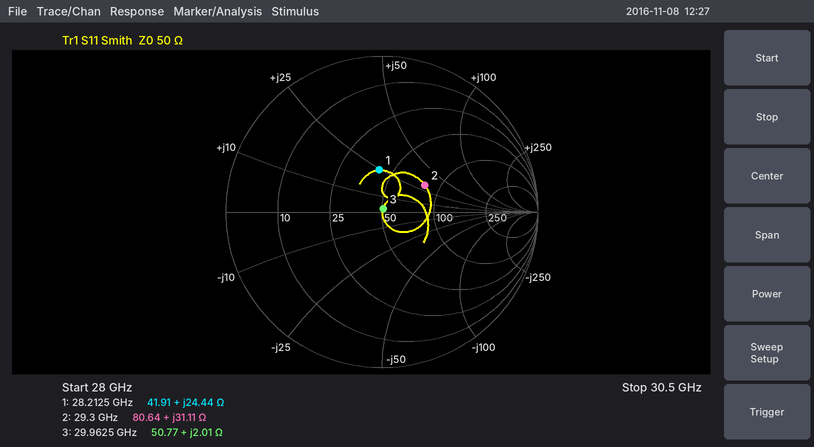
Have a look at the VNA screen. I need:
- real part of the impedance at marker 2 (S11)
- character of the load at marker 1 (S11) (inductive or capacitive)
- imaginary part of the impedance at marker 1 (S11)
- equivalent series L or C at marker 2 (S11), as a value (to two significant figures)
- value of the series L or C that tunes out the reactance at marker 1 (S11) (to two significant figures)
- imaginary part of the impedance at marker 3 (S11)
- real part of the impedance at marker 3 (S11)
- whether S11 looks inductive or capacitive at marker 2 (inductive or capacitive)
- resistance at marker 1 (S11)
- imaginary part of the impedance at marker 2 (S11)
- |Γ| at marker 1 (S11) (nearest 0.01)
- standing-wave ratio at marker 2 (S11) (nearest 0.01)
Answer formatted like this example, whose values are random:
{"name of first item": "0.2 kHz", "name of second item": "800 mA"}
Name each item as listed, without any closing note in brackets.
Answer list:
{"real part of the impedance at marker 2": "80.64 Ω", "character of the load at marker 1 (S11)": "inductive", "imaginary part of the impedance at marker 1": "+24.44 Ω", "equivalent series L or C at marker 2 (S11), as a value": "170 pH", "value of the series L or C that tunes out the reactance at marker 1 (S11)": "230 fF", "imaginary part of the impedance at marker 3": "+2.01 Ω", "real part of the impedance at marker 3": "50.77 Ω", "whether S11 looks inductive or capacitive at marker 2": "inductive", "resistance at marker 1": "41.91 Ω", "imaginary part of the impedance at marker 2": "+31.11 Ω", "|Γ| at marker 1 (S11)": "0.27", "standing-wave ratio at marker 2 (S11)": "1.96"}
